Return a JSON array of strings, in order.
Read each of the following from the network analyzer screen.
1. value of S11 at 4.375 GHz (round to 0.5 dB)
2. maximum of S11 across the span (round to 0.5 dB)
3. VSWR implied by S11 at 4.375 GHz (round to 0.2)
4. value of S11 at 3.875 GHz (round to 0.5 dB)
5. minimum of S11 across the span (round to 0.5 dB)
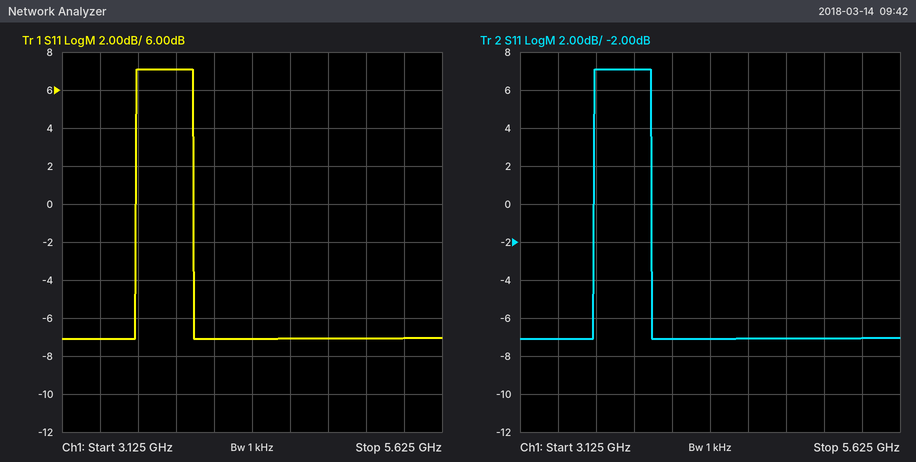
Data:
["-7.0 dB", "7.0 dB", "2.6", "7.0 dB", "-7.0 dB"]
